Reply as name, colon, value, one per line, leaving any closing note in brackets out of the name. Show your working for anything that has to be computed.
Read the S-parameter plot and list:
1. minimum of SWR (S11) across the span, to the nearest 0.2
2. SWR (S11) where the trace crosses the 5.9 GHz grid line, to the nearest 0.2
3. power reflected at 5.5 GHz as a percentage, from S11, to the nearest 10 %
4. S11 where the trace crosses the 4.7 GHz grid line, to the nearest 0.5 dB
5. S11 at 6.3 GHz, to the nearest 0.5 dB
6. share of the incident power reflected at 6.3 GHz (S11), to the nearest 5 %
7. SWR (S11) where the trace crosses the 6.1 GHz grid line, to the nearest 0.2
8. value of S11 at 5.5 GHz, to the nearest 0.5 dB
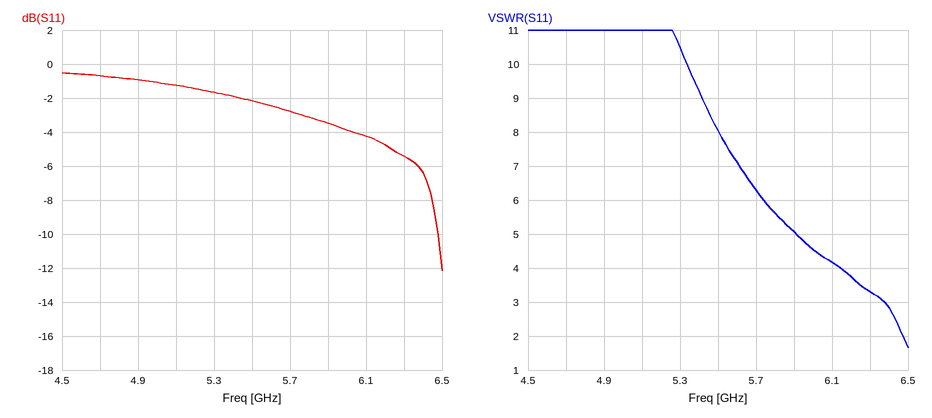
minimum of SWR (S11) across the span, to the nearest 0.2: 1.6
SWR (S11) where the trace crosses the 5.9 GHz grid line, to the nearest 0.2: 5.0
power reflected at 5.5 GHz as a percentage, from S11, to the nearest 10 %: 10^(-2/10) ≈ 63.1 %, so 60 % to the nearest 10 %
S11 where the trace crosses the 4.7 GHz grid line, to the nearest 0.5 dB: -0.5 dB
S11 at 6.3 GHz, to the nearest 0.5 dB: -5.5 dB
share of the incident power reflected at 6.3 GHz (S11), to the nearest 5 %: 10^(-5.5/10) ≈ 28.2 %, so 30 % to the nearest 5 %
SWR (S11) where the trace crosses the 6.1 GHz grid line, to the nearest 0.2: 4.2
value of S11 at 5.5 GHz, to the nearest 0.5 dB: -2.0 dB
